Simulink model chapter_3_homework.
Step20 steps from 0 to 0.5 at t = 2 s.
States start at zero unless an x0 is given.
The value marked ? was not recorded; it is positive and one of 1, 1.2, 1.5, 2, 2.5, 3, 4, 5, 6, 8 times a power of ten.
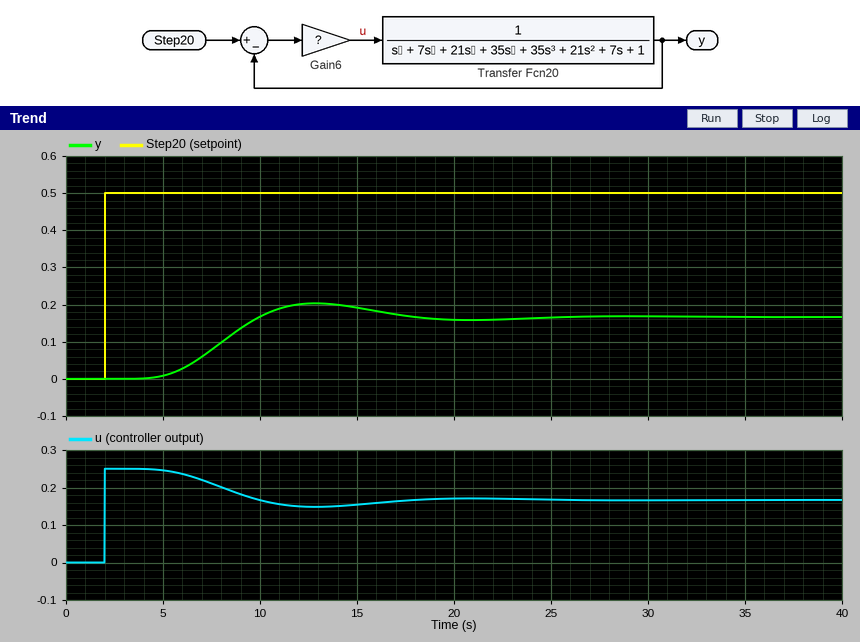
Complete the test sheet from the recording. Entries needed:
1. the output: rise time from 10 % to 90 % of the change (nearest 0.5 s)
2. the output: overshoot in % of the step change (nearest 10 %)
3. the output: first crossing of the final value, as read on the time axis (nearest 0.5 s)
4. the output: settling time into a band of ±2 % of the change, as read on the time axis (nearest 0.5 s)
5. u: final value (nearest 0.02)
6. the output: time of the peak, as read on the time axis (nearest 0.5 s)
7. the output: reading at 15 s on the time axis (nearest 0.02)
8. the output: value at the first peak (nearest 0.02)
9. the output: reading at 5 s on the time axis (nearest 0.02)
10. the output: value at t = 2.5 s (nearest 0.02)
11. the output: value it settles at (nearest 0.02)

4.0 s
20 %
10.0 s
24.0 s
0.16
13.0 s
0.20
0.20
0.00
0.00
0.16
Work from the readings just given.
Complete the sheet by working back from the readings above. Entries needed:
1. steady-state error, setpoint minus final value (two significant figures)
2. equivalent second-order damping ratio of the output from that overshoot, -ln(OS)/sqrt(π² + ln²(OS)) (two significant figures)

0.34
0.46
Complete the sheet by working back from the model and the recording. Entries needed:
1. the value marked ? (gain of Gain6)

0.5
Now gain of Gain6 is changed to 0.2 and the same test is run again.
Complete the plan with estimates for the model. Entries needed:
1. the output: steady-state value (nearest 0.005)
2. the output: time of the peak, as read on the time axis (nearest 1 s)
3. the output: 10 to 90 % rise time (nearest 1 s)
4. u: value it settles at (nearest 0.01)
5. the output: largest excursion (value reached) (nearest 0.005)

0.085
14 s
5 s
0.08
0.090
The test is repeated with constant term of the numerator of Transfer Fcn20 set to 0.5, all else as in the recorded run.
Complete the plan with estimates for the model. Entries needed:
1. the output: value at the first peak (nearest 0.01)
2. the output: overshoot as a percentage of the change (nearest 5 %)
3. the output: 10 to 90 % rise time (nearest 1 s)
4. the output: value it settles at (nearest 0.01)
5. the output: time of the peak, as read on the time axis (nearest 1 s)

0.11
10 %
5 s
0.10
14 s
